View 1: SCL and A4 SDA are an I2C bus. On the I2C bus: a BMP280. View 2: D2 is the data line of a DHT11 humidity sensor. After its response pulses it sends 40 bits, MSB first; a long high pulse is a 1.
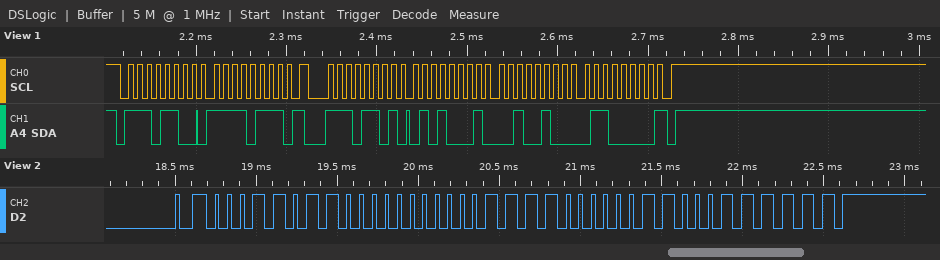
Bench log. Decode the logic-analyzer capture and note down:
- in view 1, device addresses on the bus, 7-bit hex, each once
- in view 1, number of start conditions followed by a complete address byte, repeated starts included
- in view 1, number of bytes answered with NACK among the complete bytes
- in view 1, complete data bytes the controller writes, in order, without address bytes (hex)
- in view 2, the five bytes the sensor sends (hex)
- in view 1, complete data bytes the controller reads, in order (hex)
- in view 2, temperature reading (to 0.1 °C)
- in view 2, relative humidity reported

0x76
2
1
F7
1B 00 1E 06 3F
51 24 60
30.6 °C
27 %
